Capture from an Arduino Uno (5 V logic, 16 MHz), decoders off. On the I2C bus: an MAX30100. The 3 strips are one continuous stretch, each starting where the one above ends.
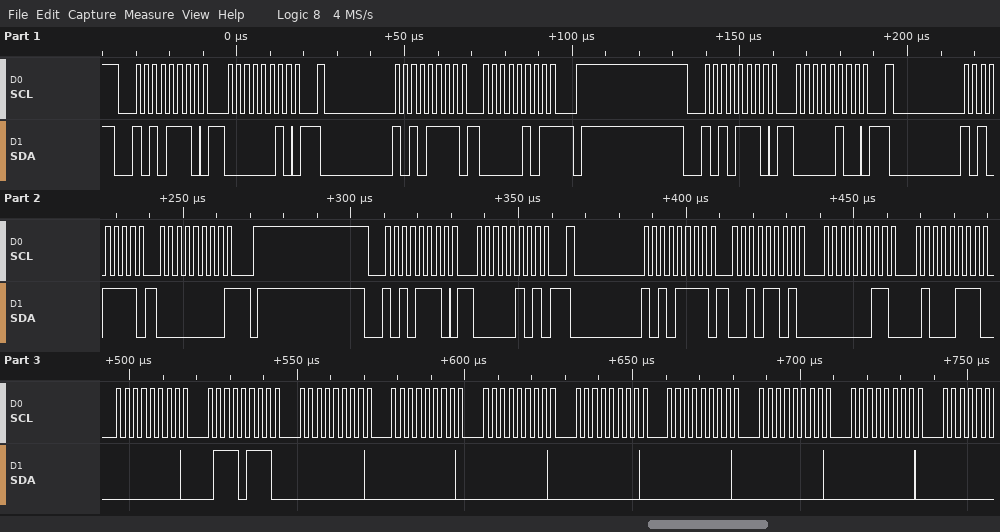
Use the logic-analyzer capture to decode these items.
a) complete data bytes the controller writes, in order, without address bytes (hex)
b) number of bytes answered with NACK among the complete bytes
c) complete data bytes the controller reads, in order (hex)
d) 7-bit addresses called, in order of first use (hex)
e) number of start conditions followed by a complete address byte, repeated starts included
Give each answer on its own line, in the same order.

02 04 05
2
05 00 2D 03 47 00 77 00 00 00 00 00 00 00
0x57
6
